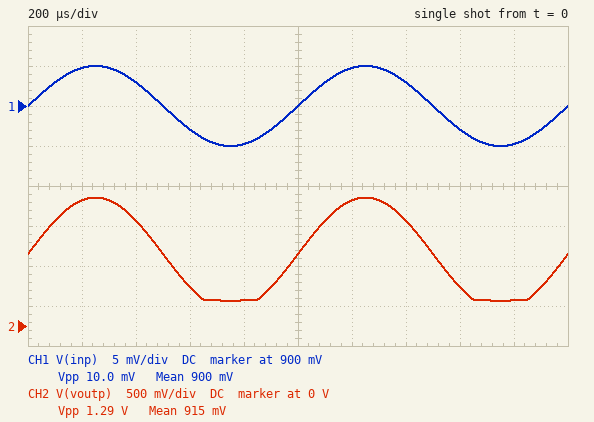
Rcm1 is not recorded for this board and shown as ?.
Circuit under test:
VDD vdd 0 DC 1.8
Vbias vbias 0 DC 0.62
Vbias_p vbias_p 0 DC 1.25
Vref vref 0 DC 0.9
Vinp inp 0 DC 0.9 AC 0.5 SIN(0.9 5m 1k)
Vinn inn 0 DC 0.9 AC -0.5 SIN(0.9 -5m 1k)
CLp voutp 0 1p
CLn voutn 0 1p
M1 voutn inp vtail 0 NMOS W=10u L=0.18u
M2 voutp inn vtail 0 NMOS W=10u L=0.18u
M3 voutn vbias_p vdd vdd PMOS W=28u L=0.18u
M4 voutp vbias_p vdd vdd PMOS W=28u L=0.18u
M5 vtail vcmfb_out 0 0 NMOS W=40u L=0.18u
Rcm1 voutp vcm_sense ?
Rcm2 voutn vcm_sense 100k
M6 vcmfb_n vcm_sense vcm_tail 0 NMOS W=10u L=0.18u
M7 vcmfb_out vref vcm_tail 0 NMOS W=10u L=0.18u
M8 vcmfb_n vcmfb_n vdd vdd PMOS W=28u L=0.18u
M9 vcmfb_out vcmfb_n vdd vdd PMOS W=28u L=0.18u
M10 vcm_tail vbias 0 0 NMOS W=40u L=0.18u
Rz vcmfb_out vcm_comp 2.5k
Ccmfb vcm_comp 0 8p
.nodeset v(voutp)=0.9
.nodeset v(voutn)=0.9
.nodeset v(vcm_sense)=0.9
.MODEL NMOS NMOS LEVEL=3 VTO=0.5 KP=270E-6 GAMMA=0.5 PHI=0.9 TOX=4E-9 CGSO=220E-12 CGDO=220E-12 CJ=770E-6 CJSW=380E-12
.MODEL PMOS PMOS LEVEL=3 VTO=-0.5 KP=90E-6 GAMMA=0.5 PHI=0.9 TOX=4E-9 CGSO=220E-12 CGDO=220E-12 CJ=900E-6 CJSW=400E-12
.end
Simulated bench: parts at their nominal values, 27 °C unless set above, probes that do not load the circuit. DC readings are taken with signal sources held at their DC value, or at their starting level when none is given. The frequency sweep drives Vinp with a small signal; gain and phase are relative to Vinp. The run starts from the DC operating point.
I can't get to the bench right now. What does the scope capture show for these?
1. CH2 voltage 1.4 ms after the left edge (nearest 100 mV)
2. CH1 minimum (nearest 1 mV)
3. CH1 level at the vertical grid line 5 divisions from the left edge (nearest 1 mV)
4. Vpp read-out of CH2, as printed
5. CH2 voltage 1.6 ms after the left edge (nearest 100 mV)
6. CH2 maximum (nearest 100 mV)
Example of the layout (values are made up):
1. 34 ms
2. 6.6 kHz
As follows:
1. 1.3 V
2. 895 mV
3. 900 mV
4. 1.29 V
5. 500 mV
6. 1.6 V
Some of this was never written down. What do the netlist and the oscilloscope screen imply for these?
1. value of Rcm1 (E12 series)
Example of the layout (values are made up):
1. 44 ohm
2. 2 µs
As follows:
1. 220 kΩ
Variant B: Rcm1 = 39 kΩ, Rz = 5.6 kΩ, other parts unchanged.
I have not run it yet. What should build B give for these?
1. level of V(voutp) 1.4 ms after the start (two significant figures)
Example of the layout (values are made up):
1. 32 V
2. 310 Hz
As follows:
1. 970 mV
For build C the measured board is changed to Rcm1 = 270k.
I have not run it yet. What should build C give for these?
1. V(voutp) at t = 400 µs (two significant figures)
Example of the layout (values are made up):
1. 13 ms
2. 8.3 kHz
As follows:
1. 1.4 V
